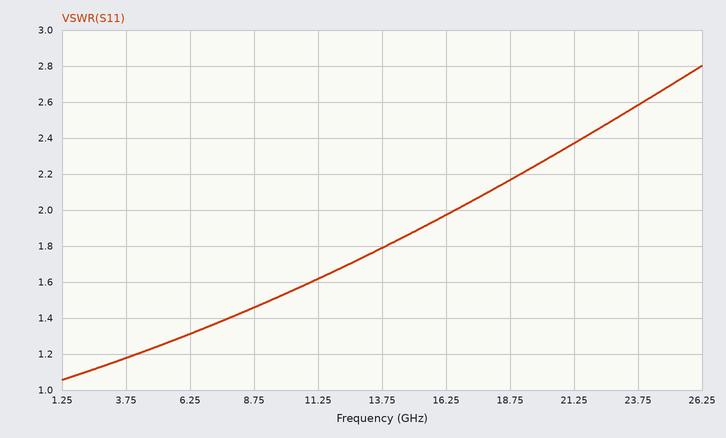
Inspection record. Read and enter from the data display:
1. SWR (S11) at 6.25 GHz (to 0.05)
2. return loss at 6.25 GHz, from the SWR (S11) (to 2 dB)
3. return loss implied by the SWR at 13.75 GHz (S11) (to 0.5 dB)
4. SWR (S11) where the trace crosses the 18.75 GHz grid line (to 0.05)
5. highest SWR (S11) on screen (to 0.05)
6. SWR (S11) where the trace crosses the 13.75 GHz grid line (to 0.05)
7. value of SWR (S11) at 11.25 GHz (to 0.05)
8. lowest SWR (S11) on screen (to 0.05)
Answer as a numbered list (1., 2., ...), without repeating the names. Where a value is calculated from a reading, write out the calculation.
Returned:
1. 1.30
2. −20 log10((1.3 − 1)/(1.3 + 1)) ≈ 18 dB
3. −20 log10((1.8 − 1)/(1.8 + 1)) ≈ 10.9 dB, so 11.0 dB to the nearest 0.5 dB
4. 2.15
5. 2.80
6. 1.80
7. 1.60
8. 1.05
